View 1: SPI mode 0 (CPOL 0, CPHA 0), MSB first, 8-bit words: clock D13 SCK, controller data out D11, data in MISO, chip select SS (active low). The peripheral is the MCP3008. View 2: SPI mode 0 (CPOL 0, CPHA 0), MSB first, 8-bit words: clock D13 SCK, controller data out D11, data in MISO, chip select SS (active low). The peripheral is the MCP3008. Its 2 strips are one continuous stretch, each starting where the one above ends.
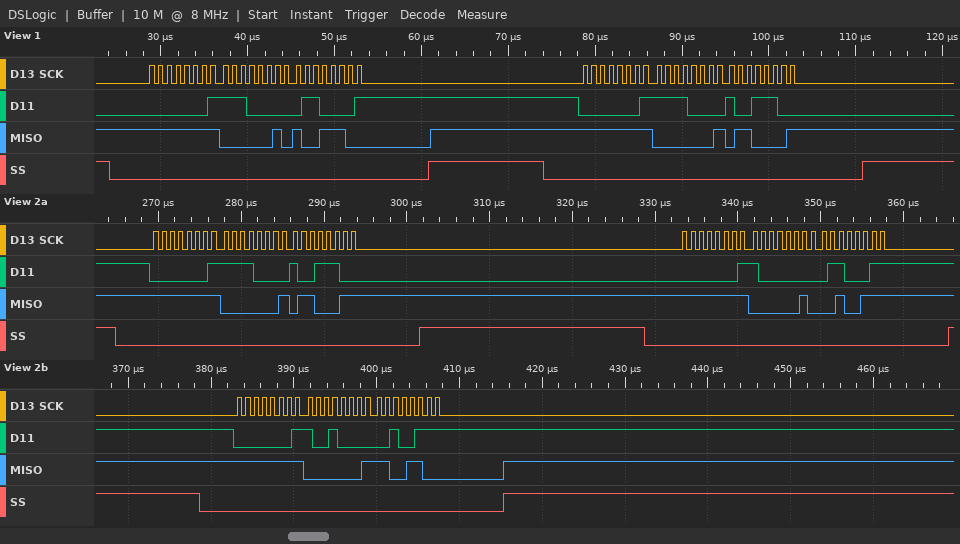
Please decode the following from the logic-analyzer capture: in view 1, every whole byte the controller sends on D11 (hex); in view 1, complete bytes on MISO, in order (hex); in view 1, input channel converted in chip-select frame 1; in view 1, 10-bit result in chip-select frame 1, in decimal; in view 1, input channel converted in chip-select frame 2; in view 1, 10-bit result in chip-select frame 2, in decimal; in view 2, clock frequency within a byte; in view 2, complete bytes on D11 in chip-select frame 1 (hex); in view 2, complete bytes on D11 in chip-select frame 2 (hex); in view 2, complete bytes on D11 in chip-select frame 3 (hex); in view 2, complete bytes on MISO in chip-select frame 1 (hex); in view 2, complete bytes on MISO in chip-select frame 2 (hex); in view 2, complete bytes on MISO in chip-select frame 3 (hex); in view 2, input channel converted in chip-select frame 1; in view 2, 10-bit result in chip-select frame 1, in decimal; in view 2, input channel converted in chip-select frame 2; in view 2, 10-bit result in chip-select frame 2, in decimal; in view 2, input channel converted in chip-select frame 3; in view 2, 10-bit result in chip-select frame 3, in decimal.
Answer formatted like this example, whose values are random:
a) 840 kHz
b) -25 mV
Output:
a) 01 E0 61 01 F0 9C
b) FF 02 9C FF 01 61
c) 6
d) 668
e) 7
f) 353
g) 1 MHz
h) 01 F0 9C
i) 01 80 63
j) 01 90 27
k) FF 01 63
l) FF 02 27
m) FF 01 CC
n) 7
o) 355
p) 0
q) 551
r) 1
s) 460
